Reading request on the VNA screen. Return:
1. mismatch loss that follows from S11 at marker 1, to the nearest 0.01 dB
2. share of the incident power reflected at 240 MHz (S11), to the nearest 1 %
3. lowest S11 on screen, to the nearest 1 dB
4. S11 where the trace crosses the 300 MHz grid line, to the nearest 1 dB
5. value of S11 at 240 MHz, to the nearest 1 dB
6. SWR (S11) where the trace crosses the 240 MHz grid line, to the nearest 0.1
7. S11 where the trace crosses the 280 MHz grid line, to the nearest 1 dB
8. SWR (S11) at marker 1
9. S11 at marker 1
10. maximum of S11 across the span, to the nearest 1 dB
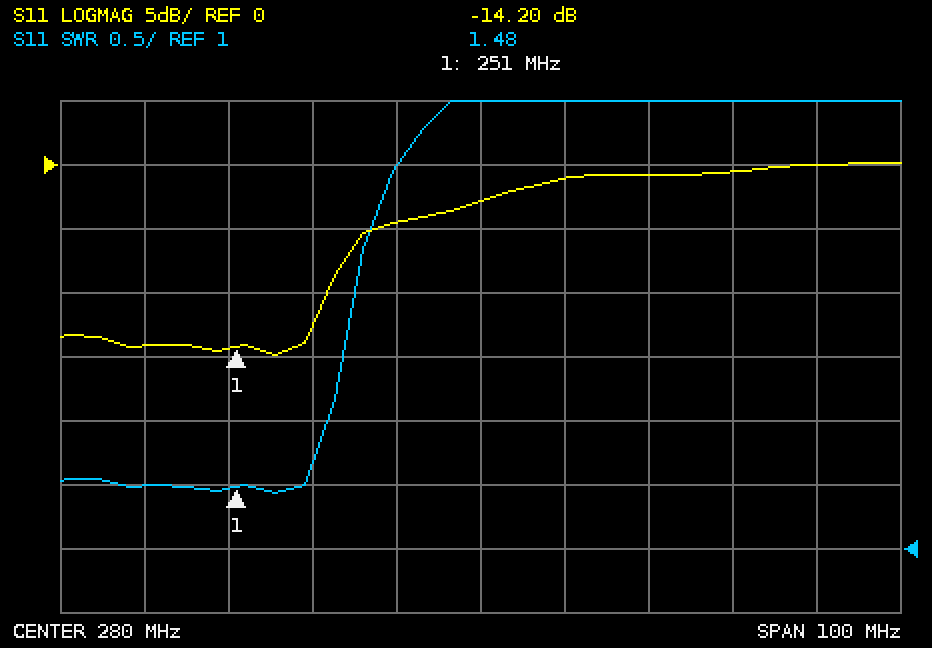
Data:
0.17 dB
4 %
-15 dB
-1 dB
-14 dB
1.5
-3 dB
1.48
-14.20 dB
0 dB
